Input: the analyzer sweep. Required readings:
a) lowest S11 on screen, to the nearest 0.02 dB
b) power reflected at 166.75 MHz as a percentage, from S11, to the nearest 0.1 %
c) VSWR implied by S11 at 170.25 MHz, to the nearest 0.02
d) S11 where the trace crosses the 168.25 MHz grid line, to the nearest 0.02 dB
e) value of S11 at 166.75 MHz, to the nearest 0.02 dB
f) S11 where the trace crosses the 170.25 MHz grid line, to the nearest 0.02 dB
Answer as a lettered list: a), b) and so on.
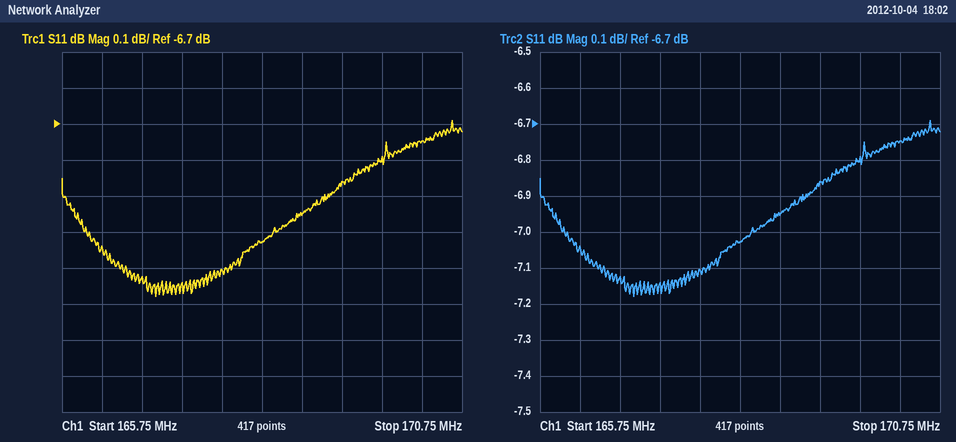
a) -7.18 dB
b) 19.4 %
c) 2.70
d) -7.02 dB
e) -7.12 dB
f) -6.74 dB
